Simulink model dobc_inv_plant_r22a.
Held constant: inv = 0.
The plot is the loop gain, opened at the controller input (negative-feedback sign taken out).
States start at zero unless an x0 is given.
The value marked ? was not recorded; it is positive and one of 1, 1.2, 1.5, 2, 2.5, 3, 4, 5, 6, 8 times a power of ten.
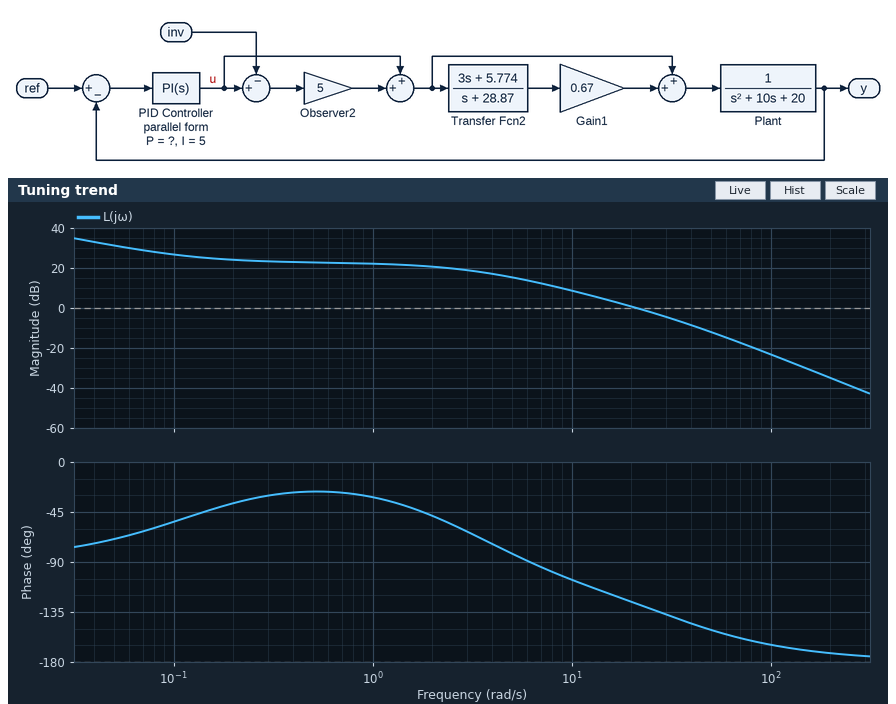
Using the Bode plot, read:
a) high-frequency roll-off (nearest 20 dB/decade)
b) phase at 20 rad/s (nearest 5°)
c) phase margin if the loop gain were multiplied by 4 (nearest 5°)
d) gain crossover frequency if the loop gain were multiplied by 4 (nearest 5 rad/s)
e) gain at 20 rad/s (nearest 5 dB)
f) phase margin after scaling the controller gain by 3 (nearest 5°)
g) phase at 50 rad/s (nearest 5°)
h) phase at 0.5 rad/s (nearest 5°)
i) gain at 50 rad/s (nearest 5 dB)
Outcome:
-40 dB/decade
-125°
30°
50 rad/s
0 dB
35°
-150°
-25°
-10 dB
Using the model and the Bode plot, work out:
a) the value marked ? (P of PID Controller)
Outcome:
40
